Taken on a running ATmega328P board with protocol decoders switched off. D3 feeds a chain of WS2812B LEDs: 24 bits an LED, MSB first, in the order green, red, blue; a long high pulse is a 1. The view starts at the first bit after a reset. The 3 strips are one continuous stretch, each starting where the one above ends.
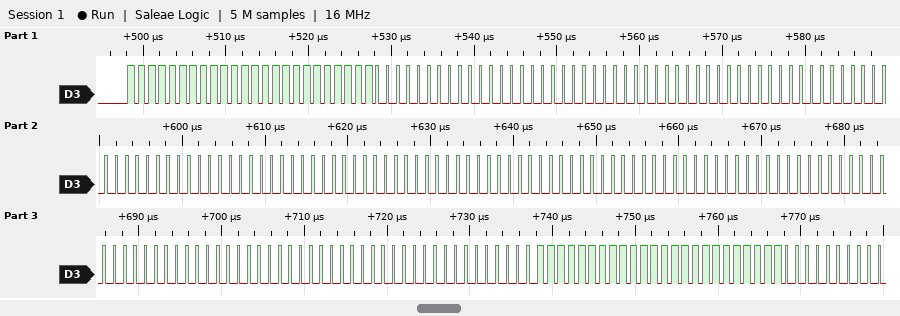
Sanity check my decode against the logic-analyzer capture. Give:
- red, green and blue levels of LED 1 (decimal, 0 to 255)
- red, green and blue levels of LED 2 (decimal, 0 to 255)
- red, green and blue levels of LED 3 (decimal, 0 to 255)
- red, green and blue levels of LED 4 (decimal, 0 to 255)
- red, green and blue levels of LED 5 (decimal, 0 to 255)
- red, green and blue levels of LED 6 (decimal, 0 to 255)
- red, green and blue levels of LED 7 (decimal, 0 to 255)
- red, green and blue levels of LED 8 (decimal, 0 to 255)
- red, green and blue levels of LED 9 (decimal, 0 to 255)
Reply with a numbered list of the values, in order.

1. 255, 255, 255
2. 0, 0, 0
3. 0, 0, 0
4. 0, 0, 0
5. 0, 0, 0
6. 0, 0, 0
7. 0, 0, 0
8. 0, 0, 0
9. 255, 255, 255
